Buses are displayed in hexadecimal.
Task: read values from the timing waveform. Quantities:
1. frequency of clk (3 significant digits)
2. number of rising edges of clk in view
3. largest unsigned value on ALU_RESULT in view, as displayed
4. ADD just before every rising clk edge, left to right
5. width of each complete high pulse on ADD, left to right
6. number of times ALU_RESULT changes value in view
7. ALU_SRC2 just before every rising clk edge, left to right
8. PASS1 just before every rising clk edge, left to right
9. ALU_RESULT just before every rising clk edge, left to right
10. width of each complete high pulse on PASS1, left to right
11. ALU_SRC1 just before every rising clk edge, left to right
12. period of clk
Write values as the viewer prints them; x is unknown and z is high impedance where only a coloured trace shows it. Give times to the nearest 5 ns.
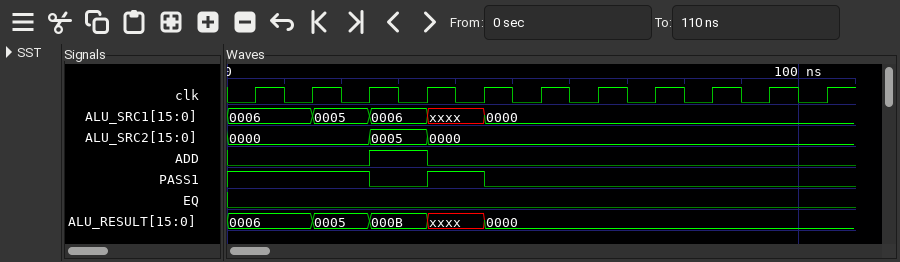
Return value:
100 MHz
11
000B
0 0 0 1 0 0 0 0 0 0 0
10 ns
4
0000, 0000, 0000, 0005, 0000, 0000, 0000, 0000, 0000, 0000, 0000
1 1 1 0 1 0 0 0 0 0 0
0006, 0006, 0005, 000B, xxxx, 0000, 0000, 0000, 0000, 0000, 0000
10 ns
0006, 0006, 0005, 0006, xxxx, 0000, 0000, 0000, 0000, 0000, 0000
10 ns
